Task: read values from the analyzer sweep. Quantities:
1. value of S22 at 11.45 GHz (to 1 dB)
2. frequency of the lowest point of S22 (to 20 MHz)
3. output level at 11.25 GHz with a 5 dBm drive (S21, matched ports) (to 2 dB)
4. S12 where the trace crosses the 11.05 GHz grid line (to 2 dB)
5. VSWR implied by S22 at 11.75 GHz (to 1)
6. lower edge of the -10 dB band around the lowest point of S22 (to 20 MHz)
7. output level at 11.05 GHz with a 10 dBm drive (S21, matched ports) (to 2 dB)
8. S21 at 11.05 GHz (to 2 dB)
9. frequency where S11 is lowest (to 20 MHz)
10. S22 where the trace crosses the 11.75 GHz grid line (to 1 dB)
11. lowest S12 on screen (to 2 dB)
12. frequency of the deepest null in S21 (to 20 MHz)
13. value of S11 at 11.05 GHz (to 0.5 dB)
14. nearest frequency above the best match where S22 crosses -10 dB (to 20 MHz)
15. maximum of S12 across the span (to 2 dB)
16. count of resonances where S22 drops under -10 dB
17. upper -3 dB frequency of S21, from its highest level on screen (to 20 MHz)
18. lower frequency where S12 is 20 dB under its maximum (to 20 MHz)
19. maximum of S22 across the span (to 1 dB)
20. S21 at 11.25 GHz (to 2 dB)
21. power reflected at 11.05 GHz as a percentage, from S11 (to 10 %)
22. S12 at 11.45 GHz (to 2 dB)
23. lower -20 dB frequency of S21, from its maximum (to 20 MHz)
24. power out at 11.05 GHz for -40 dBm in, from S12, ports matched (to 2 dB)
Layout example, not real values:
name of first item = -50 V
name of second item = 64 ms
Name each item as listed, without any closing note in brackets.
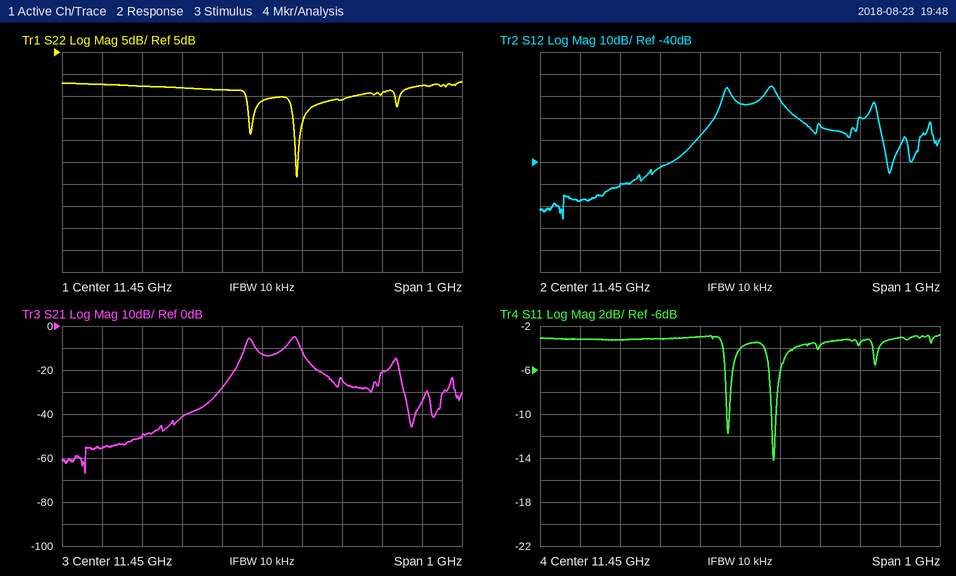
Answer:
value of S22 at 11.45 GHz = -6 dB
frequency of the lowest point of S22 = 11.54 GHz
output level at 11.25 GHz with a 5 dBm drive (S21, matched ports) = -36 dBm
S12 where the trace crosses the 11.05 GHz grid line = -58 dB
VSWR implied by S22 at 11.75 GHz = 4
lower edge of the -10 dB band around the lowest point of S22 = 11.52 GHz
output level at 11.05 GHz with a 10 dBm drive (S21, matched ports) = -46 dBm
S21 at 11.05 GHz = -56 dB
frequency where S11 is lowest = 11.54 GHz
S22 where the trace crosses the 11.75 GHz grid line = -4 dB
lowest S12 on screen = -66 dB
frequency of the deepest null in S21 = 11.00 GHz
value of S11 at 11.05 GHz = -3.0 dB
nearest frequency above the best match where S22 crosses -10 dB = 11.56 GHz
maximum of S12 across the span = -6 dB
count of resonances where S22 drops under -10 dB = 2
upper -3 dB frequency of S21, from its highest level on screen = 11.54 GHz
lower frequency where S12 is 20 dB under its maximum = 11.36 GHz
maximum of S22 across the span = -2 dB
S21 at 11.25 GHz = -42 dB
power reflected at 11.05 GHz as a percentage, from S11 = 50 %
S12 at 11.45 GHz = -14 dB
lower -20 dB frequency of S21, from its maximum = 11.36 GHz
power out at 11.05 GHz for -40 dBm in, from S12, ports matched = -98 dBm
